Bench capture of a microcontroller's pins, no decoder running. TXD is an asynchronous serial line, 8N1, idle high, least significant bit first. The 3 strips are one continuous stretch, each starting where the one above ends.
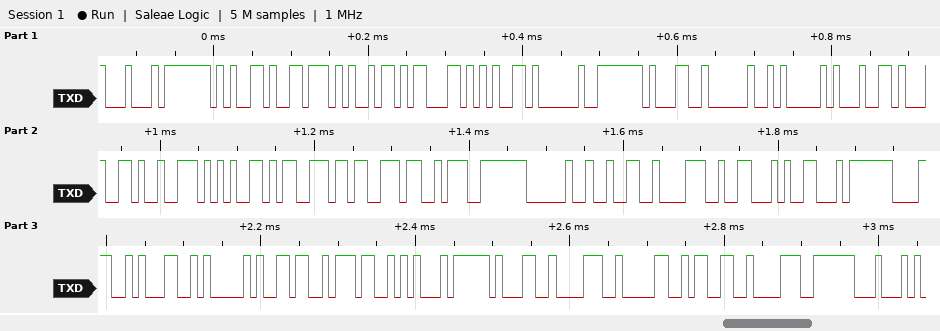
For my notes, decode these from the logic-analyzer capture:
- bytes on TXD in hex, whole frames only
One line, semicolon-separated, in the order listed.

0x44 0x65 0x76 0x69 0x63 0x65 0x20 0x31 0x20 0x41 0x64 0x64 0x72 0x65 0x73 0x73 0x3A 0x20 0x32 0x38 0x46 0x46 0x38 0x31 0x41 0x36 0x37 0x45 0x31 0x38 0x30 0x33 0x38 0x44
